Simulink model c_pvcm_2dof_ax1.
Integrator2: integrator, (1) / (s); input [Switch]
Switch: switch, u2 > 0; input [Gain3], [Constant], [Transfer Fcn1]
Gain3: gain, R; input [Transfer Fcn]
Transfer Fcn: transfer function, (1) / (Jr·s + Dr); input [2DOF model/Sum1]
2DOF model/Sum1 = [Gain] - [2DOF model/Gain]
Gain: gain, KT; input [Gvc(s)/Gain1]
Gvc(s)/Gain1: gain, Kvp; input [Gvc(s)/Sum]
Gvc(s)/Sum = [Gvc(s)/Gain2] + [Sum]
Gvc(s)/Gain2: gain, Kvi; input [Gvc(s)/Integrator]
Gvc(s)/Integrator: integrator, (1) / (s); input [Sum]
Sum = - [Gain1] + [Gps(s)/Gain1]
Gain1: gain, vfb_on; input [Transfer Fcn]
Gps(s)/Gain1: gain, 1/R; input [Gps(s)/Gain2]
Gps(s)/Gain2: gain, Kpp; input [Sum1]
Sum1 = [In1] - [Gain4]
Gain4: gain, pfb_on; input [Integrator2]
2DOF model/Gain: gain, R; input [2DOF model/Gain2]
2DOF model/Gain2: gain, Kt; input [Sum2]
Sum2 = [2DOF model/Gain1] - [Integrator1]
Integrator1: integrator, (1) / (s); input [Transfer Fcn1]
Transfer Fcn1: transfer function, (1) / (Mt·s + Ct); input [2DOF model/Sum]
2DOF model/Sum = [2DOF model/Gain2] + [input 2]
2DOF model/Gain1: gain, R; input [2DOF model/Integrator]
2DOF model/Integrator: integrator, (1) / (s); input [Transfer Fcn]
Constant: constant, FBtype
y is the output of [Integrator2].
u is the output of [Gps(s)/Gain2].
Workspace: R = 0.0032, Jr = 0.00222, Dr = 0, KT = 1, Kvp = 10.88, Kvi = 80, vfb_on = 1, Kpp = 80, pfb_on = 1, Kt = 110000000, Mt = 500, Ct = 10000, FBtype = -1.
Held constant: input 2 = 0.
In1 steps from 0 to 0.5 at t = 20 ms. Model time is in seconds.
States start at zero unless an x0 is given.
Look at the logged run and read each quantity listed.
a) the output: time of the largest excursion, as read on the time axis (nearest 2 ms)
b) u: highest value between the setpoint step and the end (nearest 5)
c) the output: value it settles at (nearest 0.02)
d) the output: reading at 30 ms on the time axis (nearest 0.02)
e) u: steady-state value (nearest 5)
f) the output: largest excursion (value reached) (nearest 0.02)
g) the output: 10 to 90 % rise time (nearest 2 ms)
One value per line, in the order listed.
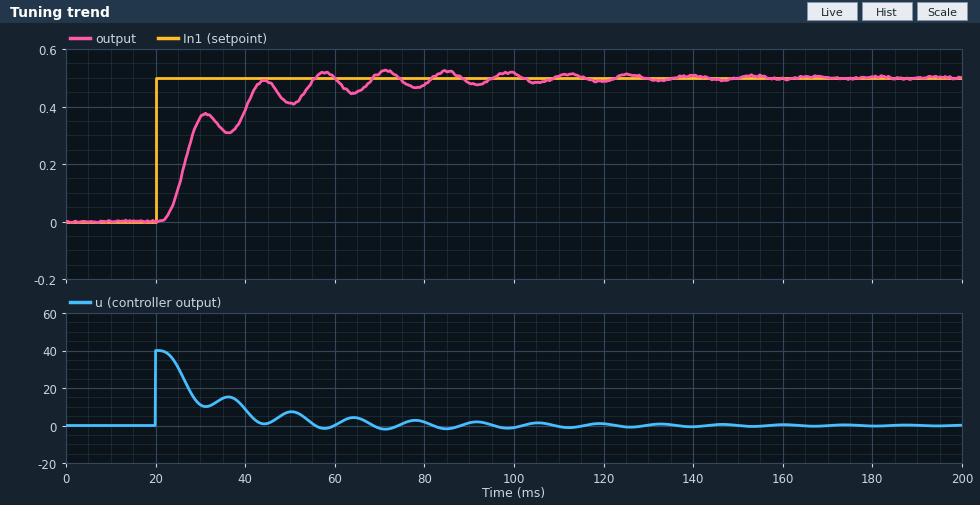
72 ms
40
0.50
0.36
0
0.52
18 ms
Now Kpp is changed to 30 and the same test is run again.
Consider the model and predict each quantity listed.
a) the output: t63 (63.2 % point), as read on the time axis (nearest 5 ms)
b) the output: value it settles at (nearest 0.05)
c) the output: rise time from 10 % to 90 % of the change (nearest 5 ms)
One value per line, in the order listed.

55 ms
0.50
70 ms
